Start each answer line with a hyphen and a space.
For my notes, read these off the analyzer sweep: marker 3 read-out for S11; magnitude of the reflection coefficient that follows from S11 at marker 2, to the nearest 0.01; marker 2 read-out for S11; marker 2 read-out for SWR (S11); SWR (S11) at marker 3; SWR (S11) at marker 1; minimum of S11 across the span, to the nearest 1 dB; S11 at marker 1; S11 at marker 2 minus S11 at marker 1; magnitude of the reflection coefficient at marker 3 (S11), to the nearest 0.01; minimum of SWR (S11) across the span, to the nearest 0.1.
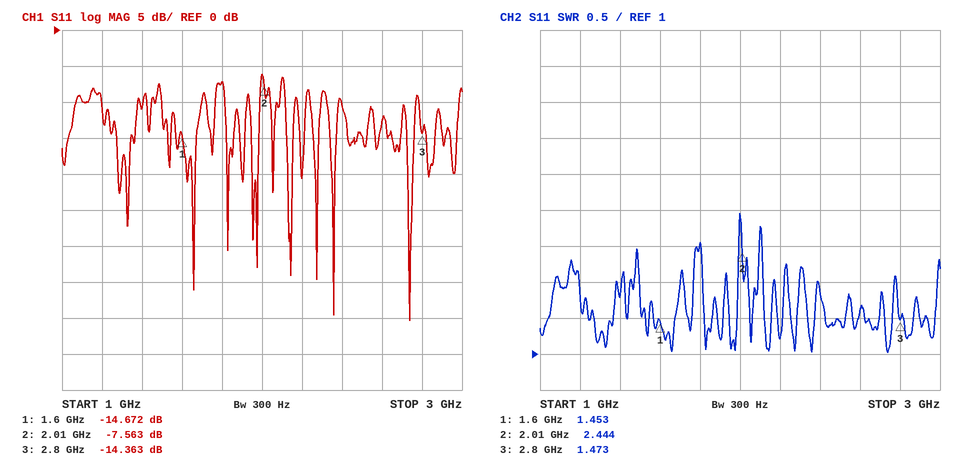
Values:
- -14.363 dB
- 0.42
- -7.563 dB
- 2.444
- 1.473
- 1.453
- -40 dB
- -14.672 dB
- 7.109 dB
- 0.19
- 1.0
